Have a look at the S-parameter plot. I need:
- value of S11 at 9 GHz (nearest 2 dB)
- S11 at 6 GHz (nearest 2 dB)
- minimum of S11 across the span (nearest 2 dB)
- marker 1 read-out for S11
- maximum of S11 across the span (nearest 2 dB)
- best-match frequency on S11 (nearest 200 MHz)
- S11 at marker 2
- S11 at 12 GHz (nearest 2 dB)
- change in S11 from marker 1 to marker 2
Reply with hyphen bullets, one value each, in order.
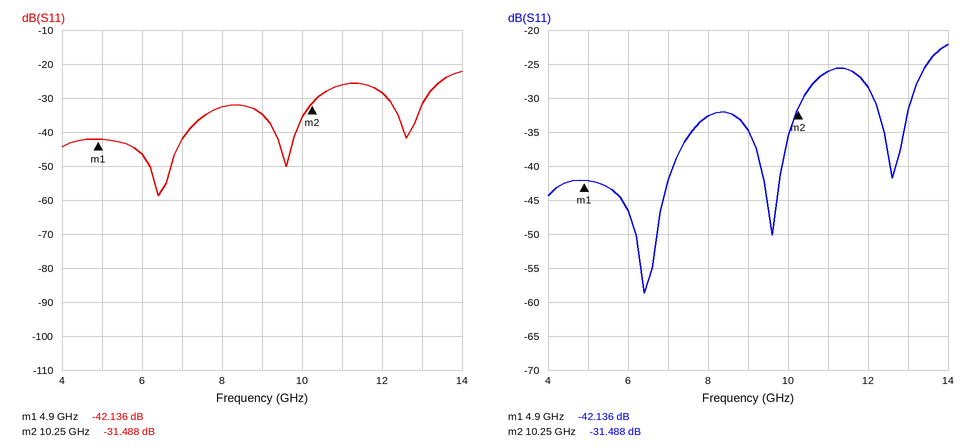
- -34 dB
- -46 dB
- -58 dB
- -42.136 dB
- -22 dB
- 6.4 GHz
- -31.488 dB
- -28 dB
- 10.648 dB
